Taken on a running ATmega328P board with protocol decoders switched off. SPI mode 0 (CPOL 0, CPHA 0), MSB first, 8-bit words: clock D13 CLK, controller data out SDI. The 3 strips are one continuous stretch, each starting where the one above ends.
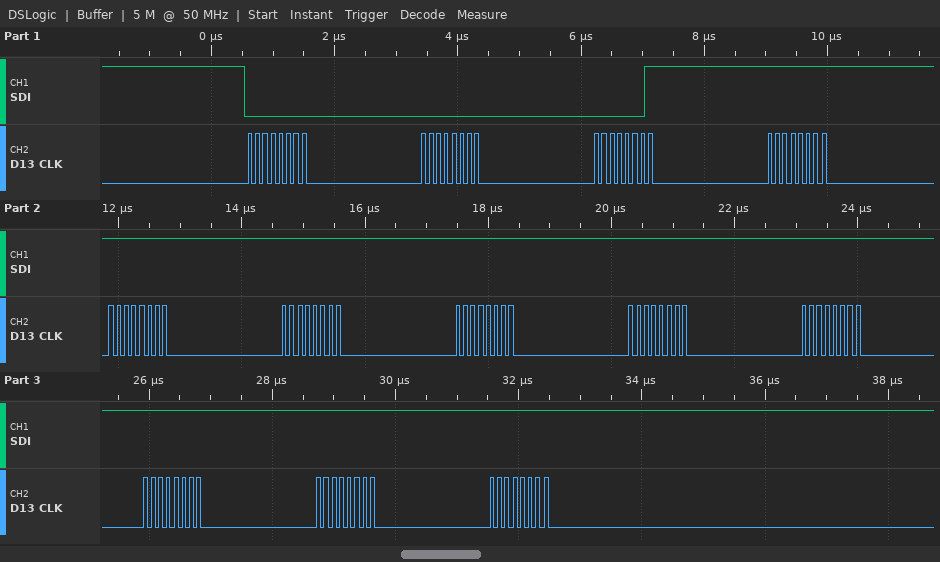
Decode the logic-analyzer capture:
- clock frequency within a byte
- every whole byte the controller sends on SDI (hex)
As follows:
8 MHz
00 00 01 FF FF FF FF FF FF FF FF FF
